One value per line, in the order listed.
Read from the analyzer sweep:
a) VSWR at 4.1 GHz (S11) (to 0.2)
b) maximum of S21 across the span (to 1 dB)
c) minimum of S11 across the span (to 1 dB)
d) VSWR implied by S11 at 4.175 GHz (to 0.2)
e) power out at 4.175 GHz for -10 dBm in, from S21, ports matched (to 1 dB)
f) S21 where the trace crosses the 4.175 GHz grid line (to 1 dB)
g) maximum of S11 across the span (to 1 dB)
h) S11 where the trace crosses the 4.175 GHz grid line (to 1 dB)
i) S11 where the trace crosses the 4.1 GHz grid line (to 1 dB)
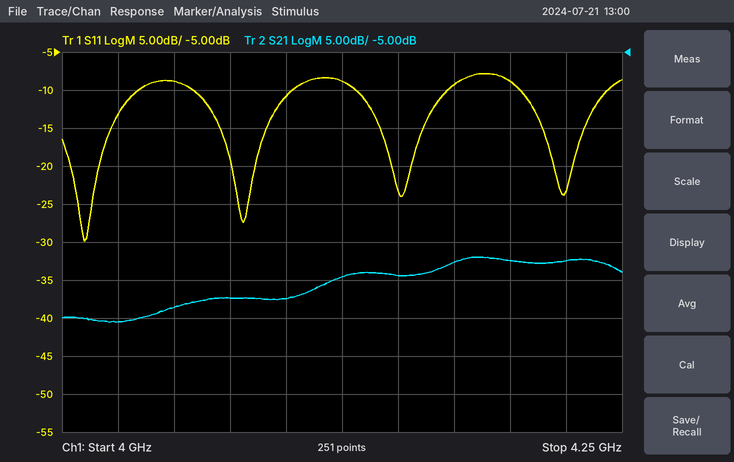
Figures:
1.8
-32 dB
-30 dB
2.0
-43 dBm
-33 dB
-8 dB
-9 dB
-11 dB
